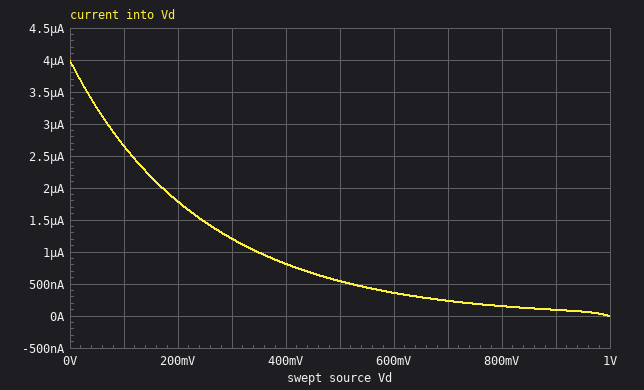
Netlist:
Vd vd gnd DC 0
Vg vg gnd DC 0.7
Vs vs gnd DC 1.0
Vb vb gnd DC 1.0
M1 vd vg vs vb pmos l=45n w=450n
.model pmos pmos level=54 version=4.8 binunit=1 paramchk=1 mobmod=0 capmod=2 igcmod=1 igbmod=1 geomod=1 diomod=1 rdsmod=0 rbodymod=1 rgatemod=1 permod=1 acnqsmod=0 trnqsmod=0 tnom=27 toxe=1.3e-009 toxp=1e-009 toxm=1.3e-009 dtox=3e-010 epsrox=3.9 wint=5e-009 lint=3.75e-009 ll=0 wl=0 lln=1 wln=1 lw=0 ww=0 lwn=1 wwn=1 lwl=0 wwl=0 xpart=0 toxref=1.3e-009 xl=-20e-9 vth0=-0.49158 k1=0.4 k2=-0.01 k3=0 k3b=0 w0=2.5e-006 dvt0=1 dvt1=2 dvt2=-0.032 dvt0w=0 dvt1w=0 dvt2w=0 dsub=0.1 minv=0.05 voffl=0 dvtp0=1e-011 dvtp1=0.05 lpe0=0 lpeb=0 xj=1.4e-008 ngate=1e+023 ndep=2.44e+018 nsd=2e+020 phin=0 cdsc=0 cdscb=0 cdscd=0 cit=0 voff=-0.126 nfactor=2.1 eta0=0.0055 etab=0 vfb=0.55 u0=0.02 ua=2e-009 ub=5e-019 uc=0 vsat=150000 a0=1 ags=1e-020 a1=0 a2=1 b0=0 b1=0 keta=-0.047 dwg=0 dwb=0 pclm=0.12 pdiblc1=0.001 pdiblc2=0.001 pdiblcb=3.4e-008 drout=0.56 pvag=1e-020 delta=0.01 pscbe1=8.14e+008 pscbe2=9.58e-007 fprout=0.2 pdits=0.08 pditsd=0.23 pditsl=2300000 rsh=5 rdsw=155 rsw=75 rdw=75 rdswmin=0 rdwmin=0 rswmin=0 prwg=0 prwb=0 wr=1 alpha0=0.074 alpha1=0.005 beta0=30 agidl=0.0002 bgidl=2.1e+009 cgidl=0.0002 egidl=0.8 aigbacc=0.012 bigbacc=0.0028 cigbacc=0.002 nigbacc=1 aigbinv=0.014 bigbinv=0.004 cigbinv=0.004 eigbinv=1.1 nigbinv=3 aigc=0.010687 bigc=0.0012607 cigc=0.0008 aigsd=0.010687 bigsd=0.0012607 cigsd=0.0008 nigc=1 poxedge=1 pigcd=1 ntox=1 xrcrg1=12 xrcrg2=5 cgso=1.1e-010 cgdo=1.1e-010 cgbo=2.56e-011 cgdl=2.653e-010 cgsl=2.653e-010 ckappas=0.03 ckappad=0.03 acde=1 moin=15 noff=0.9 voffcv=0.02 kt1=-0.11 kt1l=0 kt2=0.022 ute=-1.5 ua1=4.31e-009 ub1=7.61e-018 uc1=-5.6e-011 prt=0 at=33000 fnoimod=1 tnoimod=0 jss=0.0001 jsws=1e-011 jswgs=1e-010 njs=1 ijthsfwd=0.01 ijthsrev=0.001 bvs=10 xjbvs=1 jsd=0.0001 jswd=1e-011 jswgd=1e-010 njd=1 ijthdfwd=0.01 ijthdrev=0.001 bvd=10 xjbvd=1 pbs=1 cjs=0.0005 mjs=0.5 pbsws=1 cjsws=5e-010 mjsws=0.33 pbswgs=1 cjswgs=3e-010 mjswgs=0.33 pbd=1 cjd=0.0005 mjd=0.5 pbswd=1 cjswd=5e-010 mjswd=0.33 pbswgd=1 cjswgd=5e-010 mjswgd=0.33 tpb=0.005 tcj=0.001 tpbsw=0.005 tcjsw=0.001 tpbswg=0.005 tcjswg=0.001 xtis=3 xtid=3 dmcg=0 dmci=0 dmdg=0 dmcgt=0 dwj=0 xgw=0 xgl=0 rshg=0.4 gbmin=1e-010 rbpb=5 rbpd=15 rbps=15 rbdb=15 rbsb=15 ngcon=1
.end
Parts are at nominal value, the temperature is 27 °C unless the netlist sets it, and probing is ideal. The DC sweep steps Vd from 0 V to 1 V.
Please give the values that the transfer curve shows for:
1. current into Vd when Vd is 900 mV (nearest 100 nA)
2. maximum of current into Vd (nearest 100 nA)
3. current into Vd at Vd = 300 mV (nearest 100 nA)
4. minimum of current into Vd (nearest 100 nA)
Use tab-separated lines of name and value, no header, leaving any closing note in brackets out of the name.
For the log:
current into Vd when Vd is 900 mV	100 nA
maximum of current into Vd	4.0 µA
current into Vd at Vd = 300 mV	1.2 µA
minimum of current into Vd	0 A
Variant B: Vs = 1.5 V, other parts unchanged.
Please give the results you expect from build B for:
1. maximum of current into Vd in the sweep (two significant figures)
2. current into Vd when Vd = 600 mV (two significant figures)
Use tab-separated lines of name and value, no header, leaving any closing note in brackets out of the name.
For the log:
maximum of current into Vd in the sweep	570 µA
current into Vd when Vd = 600 mV	360 µA
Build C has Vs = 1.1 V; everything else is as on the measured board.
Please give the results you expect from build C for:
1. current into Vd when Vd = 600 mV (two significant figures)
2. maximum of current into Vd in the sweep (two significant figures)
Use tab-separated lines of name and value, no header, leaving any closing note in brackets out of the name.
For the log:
current into Vd when Vd = 600 mV	7.5 µA
maximum of current into Vd in the sweep	41 µA
